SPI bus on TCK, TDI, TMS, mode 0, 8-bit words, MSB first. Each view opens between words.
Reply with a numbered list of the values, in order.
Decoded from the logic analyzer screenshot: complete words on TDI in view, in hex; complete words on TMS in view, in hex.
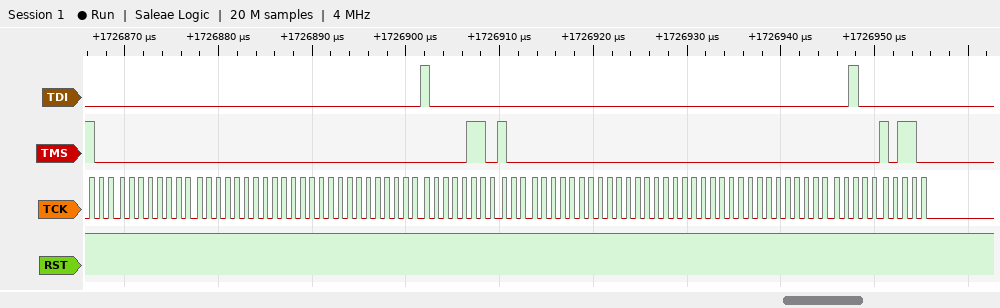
1. 00, 00, 00, 00, 10, 00, 00, 00, 00, 00, 80
2. 80, 00, 00, 00, 00, D0, 00, 00, 00, 00, 16
